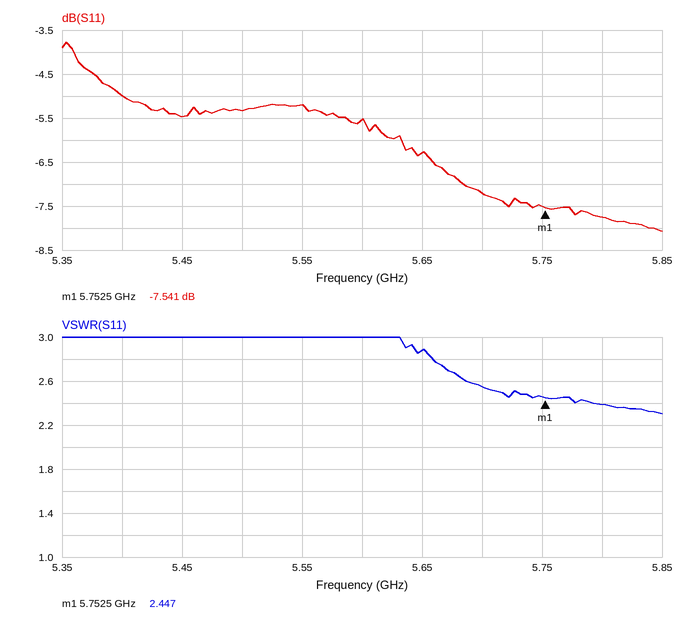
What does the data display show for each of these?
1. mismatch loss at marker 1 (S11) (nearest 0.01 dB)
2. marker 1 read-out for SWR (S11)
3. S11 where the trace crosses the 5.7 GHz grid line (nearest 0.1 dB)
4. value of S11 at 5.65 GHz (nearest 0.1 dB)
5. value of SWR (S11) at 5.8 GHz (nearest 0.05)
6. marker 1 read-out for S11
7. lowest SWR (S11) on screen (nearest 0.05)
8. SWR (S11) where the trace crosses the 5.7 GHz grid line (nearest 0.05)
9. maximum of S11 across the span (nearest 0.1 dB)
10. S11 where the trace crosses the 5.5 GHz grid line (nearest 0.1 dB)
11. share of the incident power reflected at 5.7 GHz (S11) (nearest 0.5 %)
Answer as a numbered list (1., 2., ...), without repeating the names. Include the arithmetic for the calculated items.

1. −10 log10(1 − 10^(-7.541/10)) ≈ 0.84 dB
2. 2.447
3. -7.2 dB
4. -6.3 dB
5. 2.40
6. -7.541 dB
7. 2.30
8. 2.55
9. -3.8 dB
10. -5.3 dB
11. 10^(-7.2/10) ≈ 19.1 %, so 19.0 % to the nearest 0.5 %
